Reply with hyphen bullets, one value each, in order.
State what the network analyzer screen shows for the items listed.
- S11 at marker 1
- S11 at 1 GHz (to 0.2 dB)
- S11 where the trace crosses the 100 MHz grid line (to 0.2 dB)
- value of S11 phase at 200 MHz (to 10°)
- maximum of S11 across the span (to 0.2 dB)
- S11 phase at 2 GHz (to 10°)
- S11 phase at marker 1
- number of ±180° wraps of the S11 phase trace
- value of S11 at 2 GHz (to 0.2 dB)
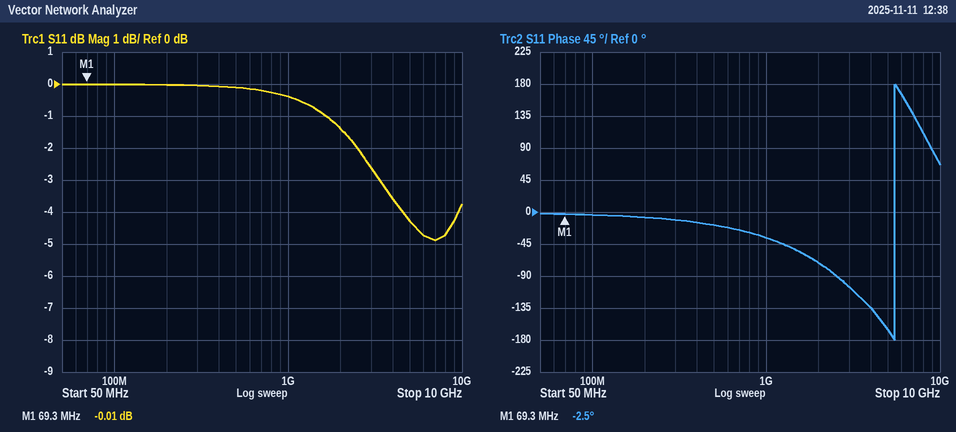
- -0.01 dB
- -0.4 dB
- 0.0 dB
- -10°
- 0.0 dB
- -70°
- -2.5°
- 1
- -1.4 dB
